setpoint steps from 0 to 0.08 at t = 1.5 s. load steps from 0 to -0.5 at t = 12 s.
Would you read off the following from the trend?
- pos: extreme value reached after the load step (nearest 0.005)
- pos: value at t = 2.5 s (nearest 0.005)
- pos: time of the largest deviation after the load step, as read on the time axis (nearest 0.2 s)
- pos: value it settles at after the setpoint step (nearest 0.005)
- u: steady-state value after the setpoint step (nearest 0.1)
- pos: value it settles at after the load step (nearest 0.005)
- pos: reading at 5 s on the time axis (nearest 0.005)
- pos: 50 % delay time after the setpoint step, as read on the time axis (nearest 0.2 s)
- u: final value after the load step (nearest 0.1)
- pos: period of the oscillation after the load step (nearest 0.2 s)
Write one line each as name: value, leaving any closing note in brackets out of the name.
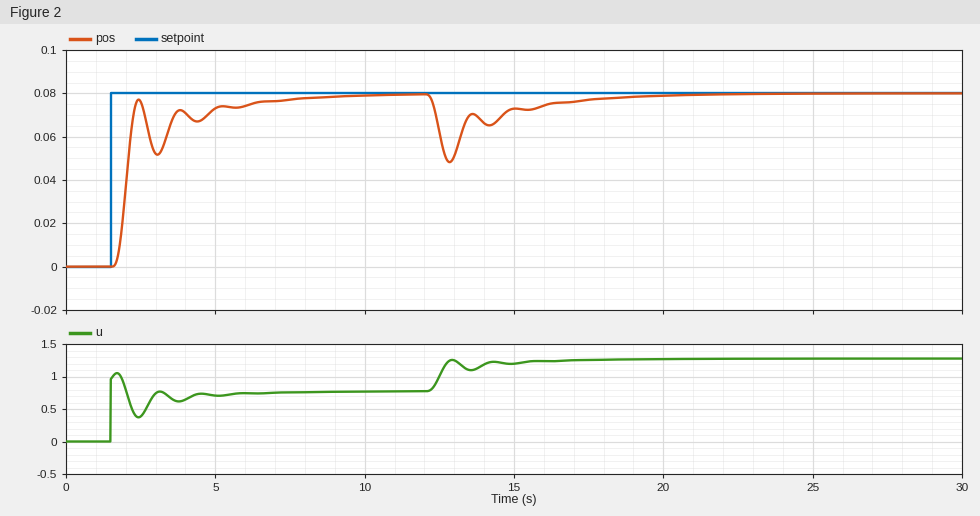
pos: extreme value reached after the load step: 0.050
pos: value at t = 2.5 s: 0.075
pos: time of the largest deviation after the load step, as read on the time axis: 12.8 s
pos: value it settles at after the setpoint step: 0.080
u: steady-state value after the setpoint step: 0.8
pos: value it settles at after the load step: 0.080
pos: reading at 5 s on the time axis: 0.075
pos: 50 % delay time after the setpoint step, as read on the time axis: 2.0 s
u: final value after the load step: 1.3
pos: period of the oscillation after the load step: 1.4 s
